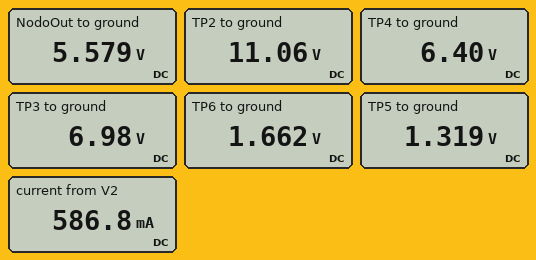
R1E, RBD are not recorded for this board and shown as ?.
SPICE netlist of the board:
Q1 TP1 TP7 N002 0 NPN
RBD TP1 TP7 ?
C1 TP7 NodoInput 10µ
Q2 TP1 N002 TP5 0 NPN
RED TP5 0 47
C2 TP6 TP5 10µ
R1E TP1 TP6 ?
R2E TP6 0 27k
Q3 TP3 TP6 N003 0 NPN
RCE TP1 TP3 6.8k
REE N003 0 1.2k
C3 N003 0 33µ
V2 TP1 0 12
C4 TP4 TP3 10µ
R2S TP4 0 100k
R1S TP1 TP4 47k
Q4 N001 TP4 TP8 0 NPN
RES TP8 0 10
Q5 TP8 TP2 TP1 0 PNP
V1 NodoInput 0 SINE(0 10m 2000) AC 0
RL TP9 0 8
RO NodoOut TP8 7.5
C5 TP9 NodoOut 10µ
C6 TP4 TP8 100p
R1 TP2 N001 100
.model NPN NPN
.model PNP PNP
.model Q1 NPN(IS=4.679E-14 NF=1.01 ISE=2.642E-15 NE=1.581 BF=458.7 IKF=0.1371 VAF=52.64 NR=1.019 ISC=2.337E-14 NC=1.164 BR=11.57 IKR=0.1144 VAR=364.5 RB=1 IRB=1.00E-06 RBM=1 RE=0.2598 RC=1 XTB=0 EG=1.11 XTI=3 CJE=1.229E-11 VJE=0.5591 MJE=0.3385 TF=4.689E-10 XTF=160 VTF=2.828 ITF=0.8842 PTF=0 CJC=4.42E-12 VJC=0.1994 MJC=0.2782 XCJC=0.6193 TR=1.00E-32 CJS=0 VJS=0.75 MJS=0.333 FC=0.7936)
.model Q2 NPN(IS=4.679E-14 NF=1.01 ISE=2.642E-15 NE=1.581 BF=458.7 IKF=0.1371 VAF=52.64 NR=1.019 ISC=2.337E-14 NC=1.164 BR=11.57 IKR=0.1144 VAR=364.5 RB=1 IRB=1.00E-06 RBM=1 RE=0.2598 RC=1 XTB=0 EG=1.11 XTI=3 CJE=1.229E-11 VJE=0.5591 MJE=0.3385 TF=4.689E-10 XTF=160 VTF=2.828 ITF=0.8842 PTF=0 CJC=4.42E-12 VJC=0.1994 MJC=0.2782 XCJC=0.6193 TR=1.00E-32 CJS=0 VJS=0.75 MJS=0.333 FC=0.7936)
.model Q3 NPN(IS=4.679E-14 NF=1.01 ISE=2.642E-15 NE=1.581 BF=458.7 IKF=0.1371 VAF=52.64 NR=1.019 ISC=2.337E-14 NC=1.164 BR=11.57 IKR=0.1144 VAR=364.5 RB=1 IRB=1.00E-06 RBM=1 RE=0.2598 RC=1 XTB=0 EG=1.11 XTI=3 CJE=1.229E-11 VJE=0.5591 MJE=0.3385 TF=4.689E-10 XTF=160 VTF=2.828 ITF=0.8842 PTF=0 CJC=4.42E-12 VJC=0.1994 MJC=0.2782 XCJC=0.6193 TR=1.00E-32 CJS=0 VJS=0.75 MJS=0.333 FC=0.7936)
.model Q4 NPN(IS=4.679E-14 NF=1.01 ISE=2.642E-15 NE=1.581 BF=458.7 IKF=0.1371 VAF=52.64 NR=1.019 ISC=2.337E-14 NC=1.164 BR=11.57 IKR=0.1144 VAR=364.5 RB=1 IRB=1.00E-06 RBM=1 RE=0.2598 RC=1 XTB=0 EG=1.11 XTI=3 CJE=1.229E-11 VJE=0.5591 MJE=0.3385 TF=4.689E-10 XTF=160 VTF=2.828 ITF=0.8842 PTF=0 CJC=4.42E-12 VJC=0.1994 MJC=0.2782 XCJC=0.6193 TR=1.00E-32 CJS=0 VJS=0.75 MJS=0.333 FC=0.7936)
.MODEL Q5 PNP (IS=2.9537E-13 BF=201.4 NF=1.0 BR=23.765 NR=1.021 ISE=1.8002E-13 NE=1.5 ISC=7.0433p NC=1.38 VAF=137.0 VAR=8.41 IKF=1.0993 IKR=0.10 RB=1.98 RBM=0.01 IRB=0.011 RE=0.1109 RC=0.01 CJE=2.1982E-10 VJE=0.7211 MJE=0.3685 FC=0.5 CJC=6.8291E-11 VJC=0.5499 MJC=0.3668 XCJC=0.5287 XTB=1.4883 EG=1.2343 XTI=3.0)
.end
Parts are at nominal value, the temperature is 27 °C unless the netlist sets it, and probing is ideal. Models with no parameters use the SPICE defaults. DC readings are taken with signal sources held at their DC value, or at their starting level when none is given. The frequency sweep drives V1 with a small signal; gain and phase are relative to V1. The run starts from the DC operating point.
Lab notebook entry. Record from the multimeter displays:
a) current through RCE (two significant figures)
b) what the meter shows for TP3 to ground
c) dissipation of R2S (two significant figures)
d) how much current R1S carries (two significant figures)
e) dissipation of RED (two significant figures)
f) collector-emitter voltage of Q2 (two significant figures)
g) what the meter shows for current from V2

740 µA
6.98 V
410 µW
120 µA
37 mW
11 V
586.8 mA
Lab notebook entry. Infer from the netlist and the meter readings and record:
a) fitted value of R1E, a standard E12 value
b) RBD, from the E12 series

150 kΩ
3.3 MΩ
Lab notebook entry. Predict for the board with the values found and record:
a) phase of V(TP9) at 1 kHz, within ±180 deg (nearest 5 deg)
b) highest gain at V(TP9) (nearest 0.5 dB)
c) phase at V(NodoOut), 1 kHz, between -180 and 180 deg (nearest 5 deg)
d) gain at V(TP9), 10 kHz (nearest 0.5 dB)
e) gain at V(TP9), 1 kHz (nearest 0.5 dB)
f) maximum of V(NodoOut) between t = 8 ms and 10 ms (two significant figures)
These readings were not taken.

-125 deg
37.0 dB
170 deg
37.0 dB
34.0 dB
6.4 V
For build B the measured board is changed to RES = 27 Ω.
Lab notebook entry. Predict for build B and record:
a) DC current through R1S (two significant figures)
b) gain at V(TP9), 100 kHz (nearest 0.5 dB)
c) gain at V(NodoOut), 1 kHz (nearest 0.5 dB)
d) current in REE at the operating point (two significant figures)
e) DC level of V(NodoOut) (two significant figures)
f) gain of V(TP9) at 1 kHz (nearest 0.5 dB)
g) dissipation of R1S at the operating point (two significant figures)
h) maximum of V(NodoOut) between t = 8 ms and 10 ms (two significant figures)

98 µA
37.5 dB
41.5 dB
750 µA
6.6 V
34.5 dB
450 µW
7.5 V
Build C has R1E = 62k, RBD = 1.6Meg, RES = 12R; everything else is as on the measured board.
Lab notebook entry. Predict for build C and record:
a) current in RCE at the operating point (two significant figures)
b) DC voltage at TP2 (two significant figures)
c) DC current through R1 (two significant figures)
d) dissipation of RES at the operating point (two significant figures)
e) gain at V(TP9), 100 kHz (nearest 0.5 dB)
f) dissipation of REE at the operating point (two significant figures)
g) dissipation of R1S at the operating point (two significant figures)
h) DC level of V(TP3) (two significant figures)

1.5 mA
11 V
4.8 mA
2.8 W
19.0 dB
2.8 mW
610 µW
1.9 V
